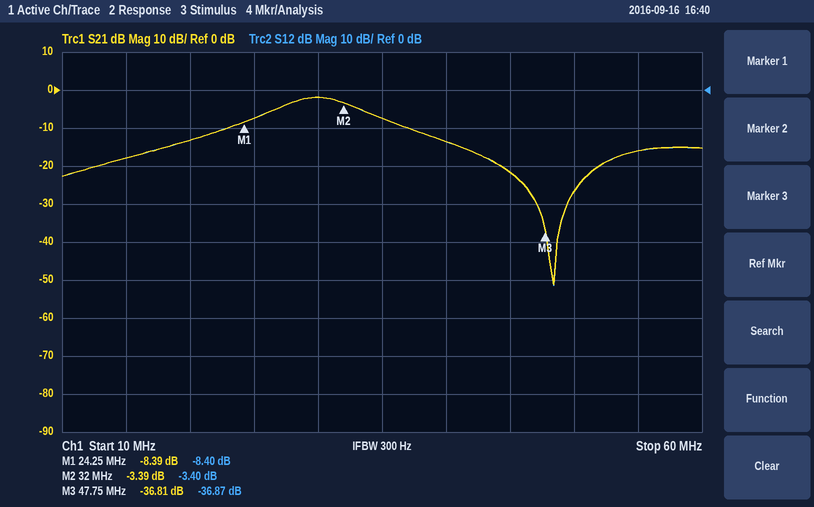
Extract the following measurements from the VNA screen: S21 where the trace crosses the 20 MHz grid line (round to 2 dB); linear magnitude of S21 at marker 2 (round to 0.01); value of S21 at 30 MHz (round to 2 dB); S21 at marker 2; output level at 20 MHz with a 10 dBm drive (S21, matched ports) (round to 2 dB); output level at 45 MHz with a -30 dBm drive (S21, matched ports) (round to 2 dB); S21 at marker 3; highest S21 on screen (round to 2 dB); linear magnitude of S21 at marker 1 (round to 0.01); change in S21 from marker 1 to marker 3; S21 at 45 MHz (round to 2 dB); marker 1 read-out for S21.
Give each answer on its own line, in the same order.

-14 dB
0.68
-2 dB
-3.39 dB
-4 dBm
-52 dBm
-36.81 dB
-2 dB
0.38
-28.42 dB
-22 dB
-8.39 dB
